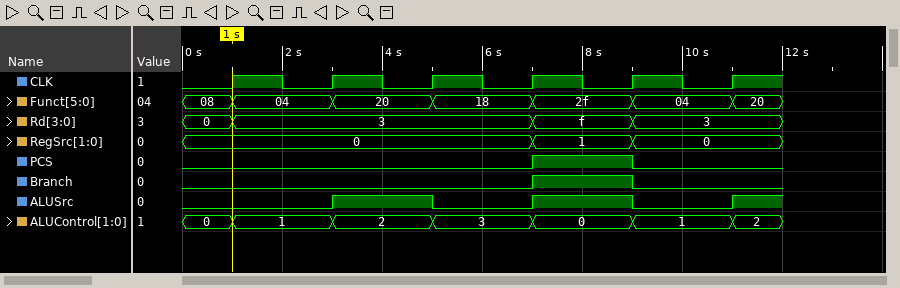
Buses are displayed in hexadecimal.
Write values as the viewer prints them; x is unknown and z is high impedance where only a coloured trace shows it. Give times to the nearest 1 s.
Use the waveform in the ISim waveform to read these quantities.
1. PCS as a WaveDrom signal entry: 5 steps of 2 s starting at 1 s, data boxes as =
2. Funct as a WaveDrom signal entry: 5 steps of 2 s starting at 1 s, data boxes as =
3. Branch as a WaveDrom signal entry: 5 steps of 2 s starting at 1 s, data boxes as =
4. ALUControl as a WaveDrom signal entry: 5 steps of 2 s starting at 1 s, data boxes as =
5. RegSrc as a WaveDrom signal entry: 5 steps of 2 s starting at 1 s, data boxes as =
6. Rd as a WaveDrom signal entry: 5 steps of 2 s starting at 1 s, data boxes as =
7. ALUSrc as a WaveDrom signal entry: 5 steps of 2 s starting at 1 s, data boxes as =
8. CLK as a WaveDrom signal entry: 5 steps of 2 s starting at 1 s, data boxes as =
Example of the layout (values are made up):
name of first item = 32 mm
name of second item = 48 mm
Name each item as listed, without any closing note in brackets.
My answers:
PCS as a WaveDrom signal entry: 5 steps of 2 s starting at 1 s, data boxes as = = {name: 'PCS', wave: '0..10'}
Funct as a WaveDrom signal entry: 5 steps of 2 s starting at 1 s, data boxes as = = {name: 'Funct', wave: '=====', data: '04 20 18 2f 04'}
Branch as a WaveDrom signal entry: 5 steps of 2 s starting at 1 s, data boxes as = = {name: 'Branch', wave: '0..10'}
ALUControl as a WaveDrom signal entry: 5 steps of 2 s starting at 1 s, data boxes as = = {name: 'ALUControl', wave: '=====', data: '1 2 3 0 1'}
RegSrc as a WaveDrom signal entry: 5 steps of 2 s starting at 1 s, data boxes as = = {name: 'RegSrc', wave: '=..==', data: '0 1 0'}
Rd as a WaveDrom signal entry: 5 steps of 2 s starting at 1 s, data boxes as = = {name: 'Rd', wave: '=..==', data: '3 f 3'}
ALUSrc as a WaveDrom signal entry: 5 steps of 2 s starting at 1 s, data boxes as = = {name: 'ALUSrc', wave: '01010'}
CLK as a WaveDrom signal entry: 5 steps of 2 s starting at 1 s, data boxes as = = {name: 'CLK', wave: 'p....'}
